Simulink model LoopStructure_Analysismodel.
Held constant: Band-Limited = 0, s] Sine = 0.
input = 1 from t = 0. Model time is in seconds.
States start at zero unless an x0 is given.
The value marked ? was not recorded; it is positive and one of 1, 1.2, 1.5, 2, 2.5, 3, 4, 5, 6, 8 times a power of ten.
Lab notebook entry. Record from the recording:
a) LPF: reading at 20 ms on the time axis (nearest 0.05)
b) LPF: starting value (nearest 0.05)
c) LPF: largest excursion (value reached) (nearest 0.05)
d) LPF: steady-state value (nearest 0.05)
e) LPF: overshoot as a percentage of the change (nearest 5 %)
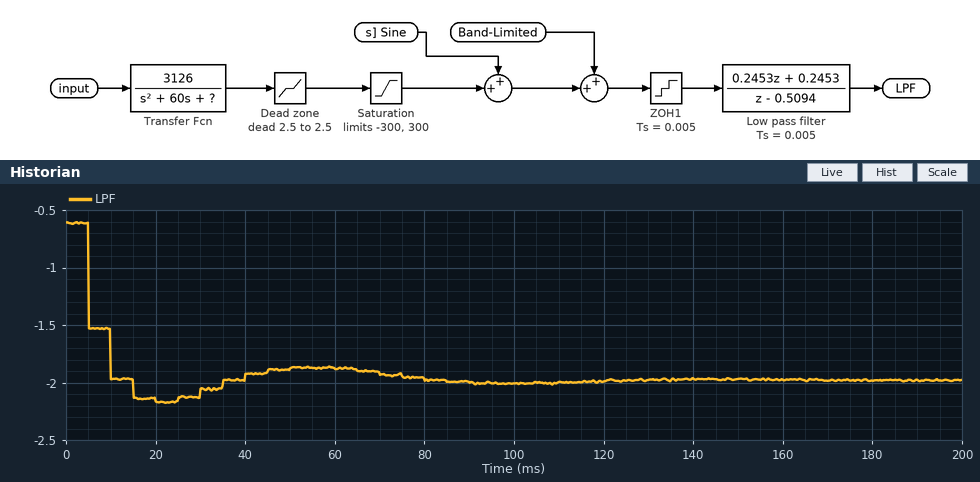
-2.15
-0.60
-2.15
-2.00
15 %
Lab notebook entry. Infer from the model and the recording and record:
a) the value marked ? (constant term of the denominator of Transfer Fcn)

6000
